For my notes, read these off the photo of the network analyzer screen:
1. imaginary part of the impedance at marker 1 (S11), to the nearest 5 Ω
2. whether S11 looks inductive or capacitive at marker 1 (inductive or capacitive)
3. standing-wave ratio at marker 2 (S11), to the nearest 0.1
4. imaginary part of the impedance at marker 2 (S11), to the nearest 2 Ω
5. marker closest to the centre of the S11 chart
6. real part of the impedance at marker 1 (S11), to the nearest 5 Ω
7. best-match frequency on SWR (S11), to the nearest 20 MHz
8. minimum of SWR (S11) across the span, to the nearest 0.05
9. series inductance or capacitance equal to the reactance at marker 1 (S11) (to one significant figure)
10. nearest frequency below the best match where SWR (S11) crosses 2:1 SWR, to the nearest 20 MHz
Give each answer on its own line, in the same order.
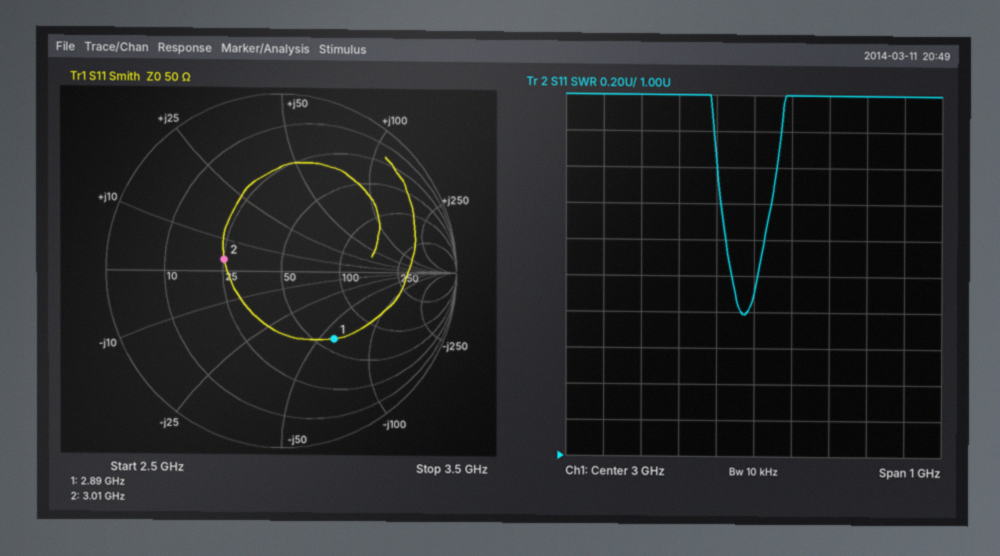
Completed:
-60 Ω
capacitive
2.0
+4 Ω
marker 2
60 Ω
2.98 GHz
1.80
900 fF
2.94 GHz
